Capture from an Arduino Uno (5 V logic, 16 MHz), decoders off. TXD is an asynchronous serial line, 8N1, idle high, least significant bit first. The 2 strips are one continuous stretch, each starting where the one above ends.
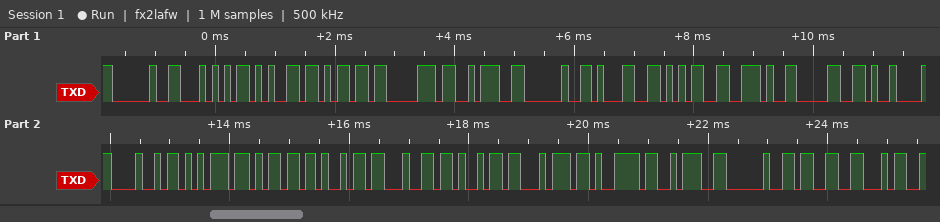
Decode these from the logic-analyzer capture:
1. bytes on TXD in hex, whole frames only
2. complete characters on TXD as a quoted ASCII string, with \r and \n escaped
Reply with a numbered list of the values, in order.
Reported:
1. 20 54 65 6D 70 3A 20 31 35 2E 30 09 48 75 6D 69 64 69 74 79 3A 20 33 34
2. " Temp: 15.0\tHumidity: 34"
